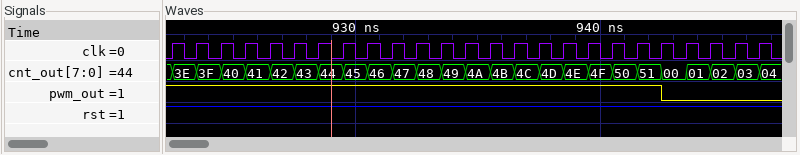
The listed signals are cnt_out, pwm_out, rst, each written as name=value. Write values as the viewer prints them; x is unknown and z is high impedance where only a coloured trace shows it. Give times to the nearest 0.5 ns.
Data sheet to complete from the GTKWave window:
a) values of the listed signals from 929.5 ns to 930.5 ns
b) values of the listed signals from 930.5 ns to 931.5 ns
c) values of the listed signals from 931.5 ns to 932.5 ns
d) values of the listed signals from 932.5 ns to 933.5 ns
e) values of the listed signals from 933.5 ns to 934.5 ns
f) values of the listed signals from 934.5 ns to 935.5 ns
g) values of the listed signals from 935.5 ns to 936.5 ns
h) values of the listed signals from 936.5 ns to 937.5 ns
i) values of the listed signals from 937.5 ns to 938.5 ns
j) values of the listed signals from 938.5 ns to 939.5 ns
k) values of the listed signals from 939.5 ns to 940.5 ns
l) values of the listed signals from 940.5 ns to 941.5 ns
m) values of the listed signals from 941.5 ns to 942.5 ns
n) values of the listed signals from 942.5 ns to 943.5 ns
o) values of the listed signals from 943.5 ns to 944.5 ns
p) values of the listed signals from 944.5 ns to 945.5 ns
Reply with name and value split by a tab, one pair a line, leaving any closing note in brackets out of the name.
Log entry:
values of the listed signals from 929.5 ns to 930.5 ns	cnt_out=45, pwm_out=1, rst=1
values of the listed signals from 930.5 ns to 931.5 ns	cnt_out=46, pwm_out=1, rst=1
values of the listed signals from 931.5 ns to 932.5 ns	cnt_out=47, pwm_out=1, rst=1
values of the listed signals from 932.5 ns to 933.5 ns	cnt_out=48, pwm_out=1, rst=1
values of the listed signals from 933.5 ns to 934.5 ns	cnt_out=49, pwm_out=1, rst=1
values of the listed signals from 934.5 ns to 935.5 ns	cnt_out=4A, pwm_out=1, rst=1
values of the listed signals from 935.5 ns to 936.5 ns	cnt_out=4B, pwm_out=1, rst=1
values of the listed signals from 936.5 ns to 937.5 ns	cnt_out=4C, pwm_out=1, rst=1
values of the listed signals from 937.5 ns to 938.5 ns	cnt_out=4D, pwm_out=1, rst=1
values of the listed signals from 938.5 ns to 939.5 ns	cnt_out=4E, pwm_out=1, rst=1
values of the listed signals from 939.5 ns to 940.5 ns	cnt_out=4F, pwm_out=1, rst=1
values of the listed signals from 940.5 ns to 941.5 ns	cnt_out=50, pwm_out=1, rst=1
values of the listed signals from 941.5 ns to 942.5 ns	cnt_out=51, pwm_out=1, rst=1
values of the listed signals from 942.5 ns to 943.5 ns	cnt_out=00, pwm_out=0, rst=1
values of the listed signals from 943.5 ns to 944.5 ns	cnt_out=01, pwm_out=0, rst=1
values of the listed signals from 944.5 ns to 945.5 ns	cnt_out=02, pwm_out=0, rst=1
